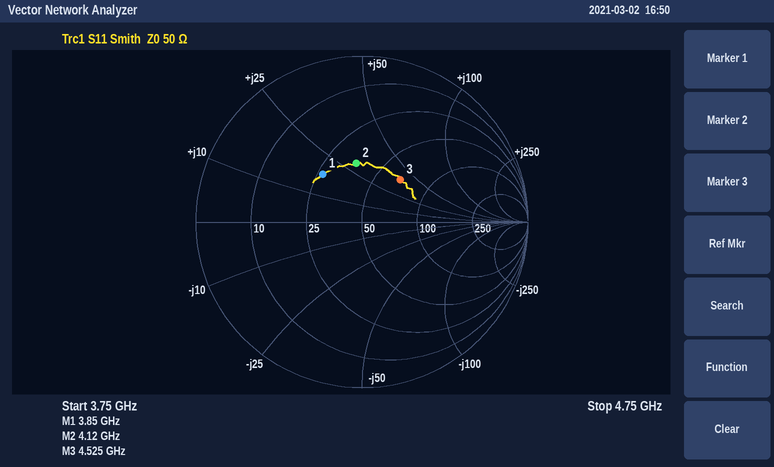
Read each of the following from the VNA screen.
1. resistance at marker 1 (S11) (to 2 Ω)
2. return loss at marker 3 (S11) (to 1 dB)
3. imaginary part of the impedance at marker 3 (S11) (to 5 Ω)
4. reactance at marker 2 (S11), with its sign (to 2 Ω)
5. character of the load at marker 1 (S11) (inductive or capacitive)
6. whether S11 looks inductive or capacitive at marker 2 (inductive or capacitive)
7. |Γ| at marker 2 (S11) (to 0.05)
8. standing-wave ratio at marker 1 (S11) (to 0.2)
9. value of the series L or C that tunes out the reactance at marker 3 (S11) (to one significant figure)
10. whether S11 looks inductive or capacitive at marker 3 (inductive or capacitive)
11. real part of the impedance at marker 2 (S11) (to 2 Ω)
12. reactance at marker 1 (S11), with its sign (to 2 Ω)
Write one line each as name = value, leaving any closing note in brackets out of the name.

resistance at marker 1 (S11) = 26 Ω
return loss at marker 3 (S11) = 9 dB
imaginary part of the impedance at marker 3 (S11) = +40 Ω
reactance at marker 2 (S11), with its sign = +30 Ω
character of the load at marker 1 (S11) = inductive
whether S11 looks inductive or capacitive at marker 2 = inductive
|Γ| at marker 2 (S11) = 0.35
standing-wave ratio at marker 1 (S11) = 2.2
value of the series L or C that tunes out the reactance at marker 3 (S11) = 900 fF
whether S11 looks inductive or capacitive at marker 3 = inductive
real part of the impedance at marker 2 (S11) = 36 Ω
reactance at marker 1 (S11), with its sign = +18 Ω
